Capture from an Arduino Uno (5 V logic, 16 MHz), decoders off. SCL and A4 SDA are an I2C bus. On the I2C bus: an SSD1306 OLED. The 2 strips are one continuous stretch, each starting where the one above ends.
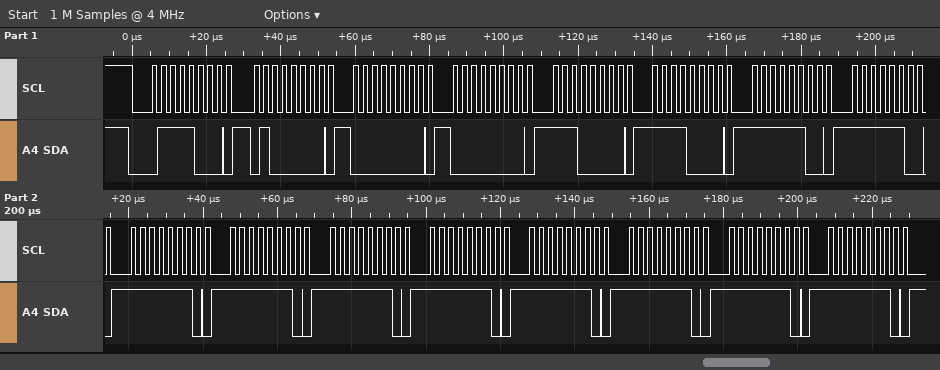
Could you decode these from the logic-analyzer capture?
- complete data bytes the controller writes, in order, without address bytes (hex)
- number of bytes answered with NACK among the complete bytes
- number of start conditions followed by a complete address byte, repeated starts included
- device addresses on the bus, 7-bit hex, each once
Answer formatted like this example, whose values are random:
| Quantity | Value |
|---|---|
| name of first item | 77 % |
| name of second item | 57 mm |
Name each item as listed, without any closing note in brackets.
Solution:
| Quantity | Value |
|---|---|
| complete data bytes the controller writes, in order, without address bytes | 40 00 00 E0 F0 FC FC FE FE FE FE FE FE FE FE |
| number of bytes answered with NACK among the complete bytes | 0 |
| number of start conditions followed by a complete address byte, repeated starts included | 1 |
| device addresses on the bus, 7-bit hex, each once | 0x3C |
